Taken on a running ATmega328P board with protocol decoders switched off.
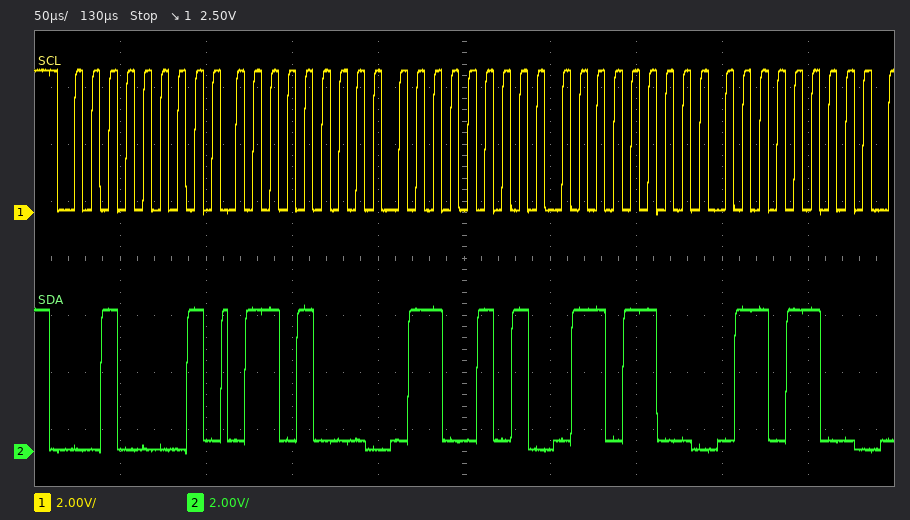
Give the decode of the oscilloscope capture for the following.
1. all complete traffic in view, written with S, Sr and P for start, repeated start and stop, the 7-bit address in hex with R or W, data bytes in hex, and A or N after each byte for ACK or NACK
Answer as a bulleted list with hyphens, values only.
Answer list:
- S 10R A 68 A 65 A 6C A 6C A
